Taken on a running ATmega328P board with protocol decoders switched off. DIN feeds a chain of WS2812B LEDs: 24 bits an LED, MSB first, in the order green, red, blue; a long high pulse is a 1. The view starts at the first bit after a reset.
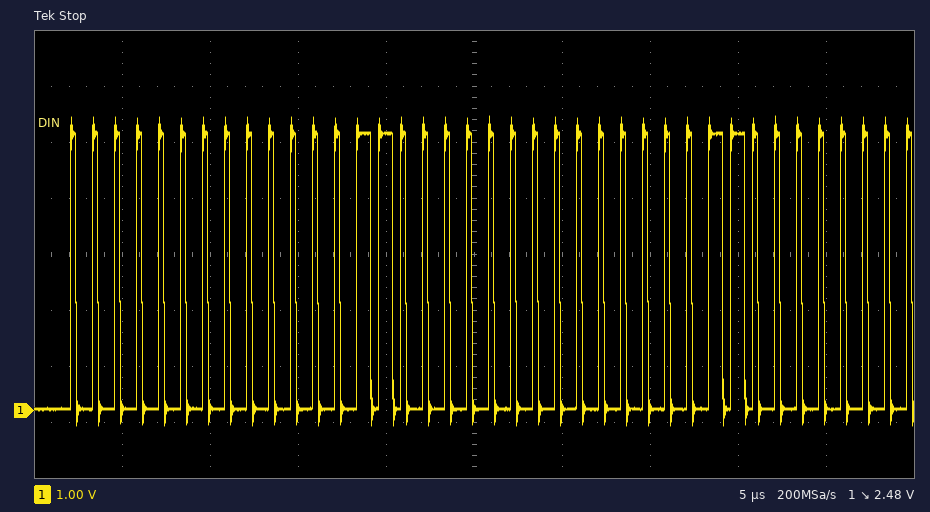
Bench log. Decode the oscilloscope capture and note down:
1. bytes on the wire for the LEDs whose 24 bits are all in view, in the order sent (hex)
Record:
00 06 00
